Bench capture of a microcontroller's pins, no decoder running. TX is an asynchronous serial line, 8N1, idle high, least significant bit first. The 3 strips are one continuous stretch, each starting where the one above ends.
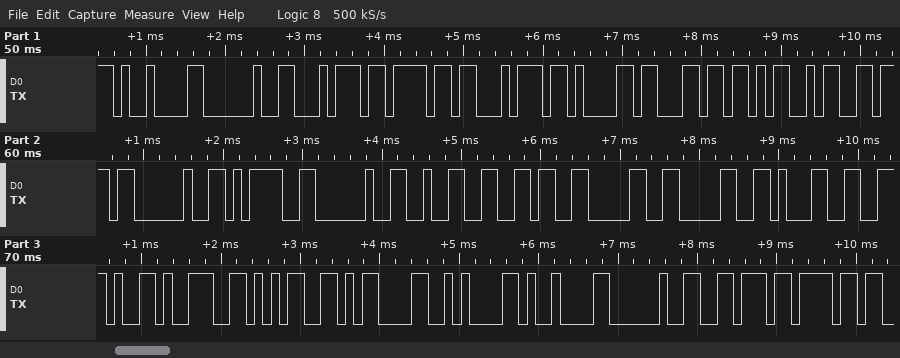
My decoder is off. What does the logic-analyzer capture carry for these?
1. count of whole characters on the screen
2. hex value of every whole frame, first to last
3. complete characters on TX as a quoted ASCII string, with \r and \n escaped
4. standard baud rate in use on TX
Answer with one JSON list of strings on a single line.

["26", "0x09 0x20 0x74 0x6F 0x74 0x61 0x6C 0x4D 0x76 0x20 0x3D 0x20 0x32 0x36 0x30 0x30 0x31 0x2E 0x39 0x35 0x0D 0x0A 0x09 0x20 0x76 0x6F", "\"\\t totalMv = 26001.95\\r\\n\\t vo\"", "9600 baud"]
